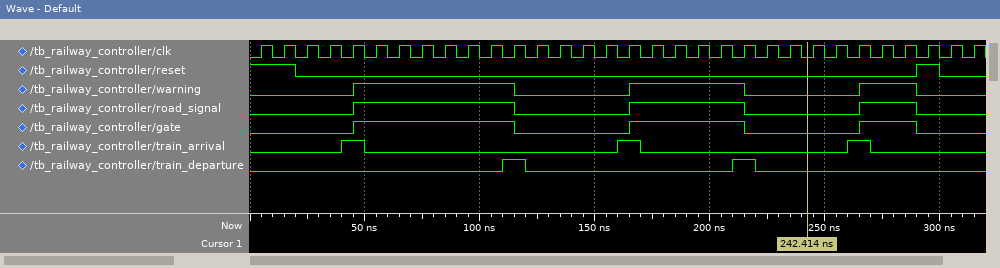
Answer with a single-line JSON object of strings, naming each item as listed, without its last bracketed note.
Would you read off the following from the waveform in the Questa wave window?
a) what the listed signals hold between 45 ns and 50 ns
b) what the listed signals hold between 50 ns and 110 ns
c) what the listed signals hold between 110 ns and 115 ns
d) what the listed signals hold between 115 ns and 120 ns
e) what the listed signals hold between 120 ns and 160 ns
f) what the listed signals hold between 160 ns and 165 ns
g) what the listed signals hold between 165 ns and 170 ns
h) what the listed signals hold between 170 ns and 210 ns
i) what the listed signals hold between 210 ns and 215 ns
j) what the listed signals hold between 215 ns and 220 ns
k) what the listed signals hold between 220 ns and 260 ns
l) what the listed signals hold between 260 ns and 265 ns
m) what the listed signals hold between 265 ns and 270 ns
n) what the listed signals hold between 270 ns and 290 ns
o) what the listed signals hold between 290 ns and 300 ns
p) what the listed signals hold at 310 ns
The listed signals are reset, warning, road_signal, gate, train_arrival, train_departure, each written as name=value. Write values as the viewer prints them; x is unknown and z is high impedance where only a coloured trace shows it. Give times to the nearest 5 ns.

{"what the listed signals hold between 45 ns and 50 ns": "reset=0, warning=1, road_signal=1, gate=1, train_arrival=1, train_departure=0", "what the listed signals hold between 50 ns and 110 ns": "reset=0, warning=1, road_signal=1, gate=1, train_arrival=0, train_departure=0", "what the listed signals hold between 110 ns and 115 ns": "reset=0, warning=1, road_signal=1, gate=1, train_arrival=0, train_departure=1", "what the listed signals hold between 115 ns and 120 ns": "reset=0, warning=0, road_signal=0, gate=0, train_arrival=0, train_departure=1", "what the listed signals hold between 120 ns and 160 ns": "reset=0, warning=0, road_signal=0, gate=0, train_arrival=0, train_departure=0", "what the listed signals hold between 160 ns and 165 ns": "reset=0, warning=0, road_signal=0, gate=0, train_arrival=1, train_departure=0", "what the listed signals hold between 165 ns and 170 ns": "reset=0, warning=1, road_signal=1, gate=1, train_arrival=1, train_departure=0", "what the listed signals hold between 170 ns and 210 ns": "reset=0, warning=1, road_signal=1, gate=1, train_arrival=0, train_departure=0", "what the listed signals hold between 210 ns and 215 ns": "reset=0, warning=1, road_signal=1, gate=1, train_arrival=0, train_departure=1", "what the listed signals hold between 215 ns and 220 ns": "reset=0, warning=0, road_signal=0, gate=0, train_arrival=0, train_departure=1", "what the listed signals hold between 220 ns and 260 ns": "reset=0, warning=0, road_signal=0, gate=0, train_arrival=0, train_departure=0", "what the listed signals hold between 260 ns and 265 ns": "reset=0, warning=0, road_signal=0, gate=0, train_arrival=1, train_departure=0", "what the listed signals hold between 265 ns and 270 ns": "reset=0, warning=1, road_signal=1, gate=1, train_arrival=1, train_departure=0", "what the listed signals hold between 270 ns and 290 ns": "reset=0, warning=1, road_signal=1, gate=1, train_arrival=0, train_departure=0", "what the listed signals hold between 290 ns and 300 ns": "reset=1, warning=0, road_signal=0, gate=0, train_arrival=0, train_departure=0", "what the listed signals hold at 310 ns": "reset=0, warning=0, road_signal=0, gate=0, train_arrival=0, train_departure=0"}
